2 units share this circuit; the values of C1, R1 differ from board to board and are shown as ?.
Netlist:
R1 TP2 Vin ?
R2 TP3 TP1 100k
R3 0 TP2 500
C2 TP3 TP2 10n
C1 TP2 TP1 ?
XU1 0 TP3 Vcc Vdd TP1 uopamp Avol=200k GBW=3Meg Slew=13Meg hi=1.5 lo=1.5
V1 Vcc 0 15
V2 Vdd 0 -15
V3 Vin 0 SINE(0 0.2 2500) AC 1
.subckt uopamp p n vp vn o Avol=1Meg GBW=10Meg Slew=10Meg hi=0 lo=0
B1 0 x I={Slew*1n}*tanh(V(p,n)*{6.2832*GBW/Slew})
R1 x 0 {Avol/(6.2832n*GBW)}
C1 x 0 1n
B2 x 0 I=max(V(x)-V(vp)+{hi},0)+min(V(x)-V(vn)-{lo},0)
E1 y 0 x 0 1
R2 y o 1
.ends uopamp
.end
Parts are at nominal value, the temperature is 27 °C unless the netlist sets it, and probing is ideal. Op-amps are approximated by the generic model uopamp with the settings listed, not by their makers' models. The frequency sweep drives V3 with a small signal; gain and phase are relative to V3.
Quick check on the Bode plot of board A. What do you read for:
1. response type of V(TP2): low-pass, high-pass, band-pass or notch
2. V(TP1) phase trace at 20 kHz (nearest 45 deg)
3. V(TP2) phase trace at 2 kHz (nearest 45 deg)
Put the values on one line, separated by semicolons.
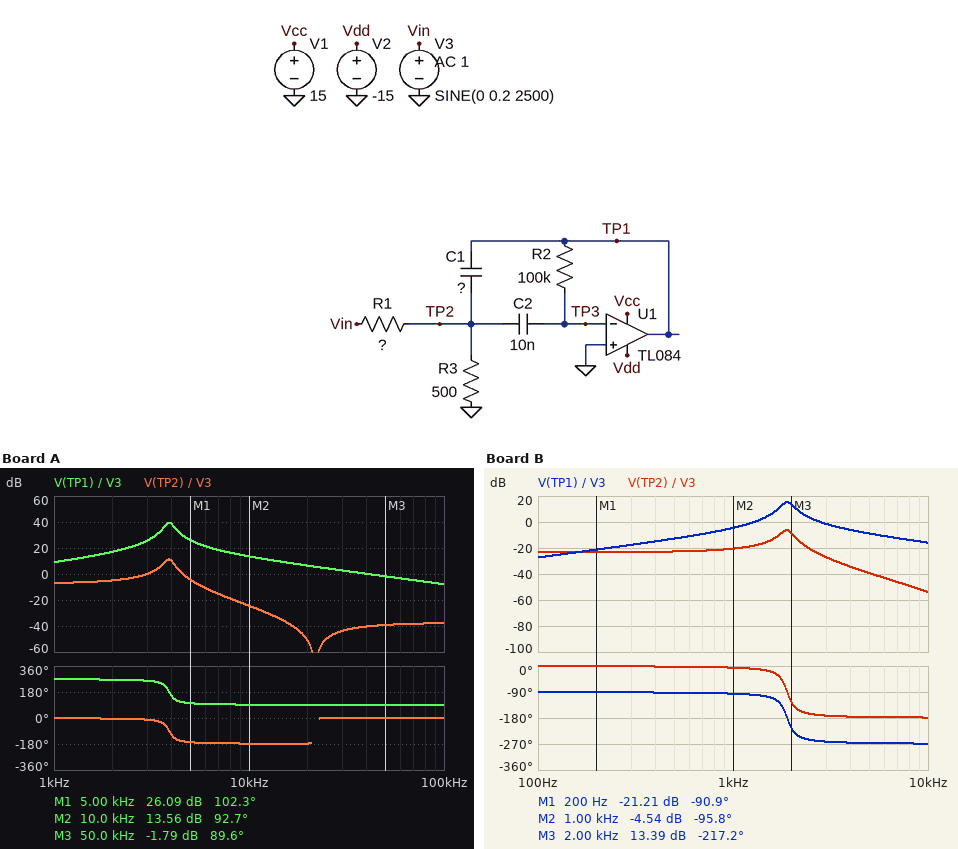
band-pass; 90 deg; 0 deg
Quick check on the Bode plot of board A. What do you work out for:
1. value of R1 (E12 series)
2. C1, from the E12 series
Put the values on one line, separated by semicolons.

680 Ω; 5.6 nF
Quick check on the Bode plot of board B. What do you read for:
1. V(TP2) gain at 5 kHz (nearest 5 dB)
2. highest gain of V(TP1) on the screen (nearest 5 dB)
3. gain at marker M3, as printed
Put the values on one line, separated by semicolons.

-40 dB; 15 dB; 13.39 dB
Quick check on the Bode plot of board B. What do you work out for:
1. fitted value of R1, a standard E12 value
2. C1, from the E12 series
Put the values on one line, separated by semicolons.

6.8 kΩ; 15 nF
